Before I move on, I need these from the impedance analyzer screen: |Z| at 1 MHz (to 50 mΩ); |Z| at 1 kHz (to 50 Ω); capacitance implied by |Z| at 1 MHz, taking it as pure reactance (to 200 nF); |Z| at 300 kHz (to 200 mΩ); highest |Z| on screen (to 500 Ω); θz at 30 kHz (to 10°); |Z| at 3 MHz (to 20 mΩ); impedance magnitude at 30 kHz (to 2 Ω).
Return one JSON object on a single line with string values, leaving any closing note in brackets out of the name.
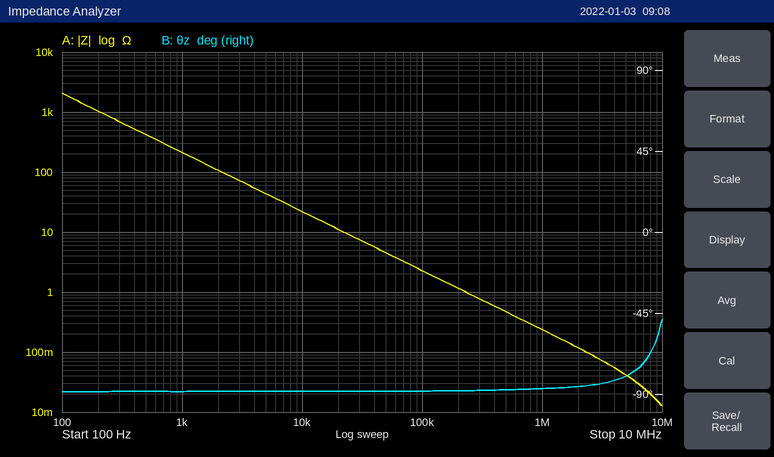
{"|Z| at 1 MHz": "250 mΩ", "|Z| at 1 kHz": "200 Ω", "capacitance implied by |Z| at 1 MHz, taking it as pure reactance": "600 nF", "|Z| at 300 kHz": "800 mΩ", "highest |Z| on screen": "2.0 kΩ", "θz at 30 kHz": "-90°", "|Z| at 3 MHz": "80 mΩ", "impedance magnitude at 30 kHz": "8 Ω"}
